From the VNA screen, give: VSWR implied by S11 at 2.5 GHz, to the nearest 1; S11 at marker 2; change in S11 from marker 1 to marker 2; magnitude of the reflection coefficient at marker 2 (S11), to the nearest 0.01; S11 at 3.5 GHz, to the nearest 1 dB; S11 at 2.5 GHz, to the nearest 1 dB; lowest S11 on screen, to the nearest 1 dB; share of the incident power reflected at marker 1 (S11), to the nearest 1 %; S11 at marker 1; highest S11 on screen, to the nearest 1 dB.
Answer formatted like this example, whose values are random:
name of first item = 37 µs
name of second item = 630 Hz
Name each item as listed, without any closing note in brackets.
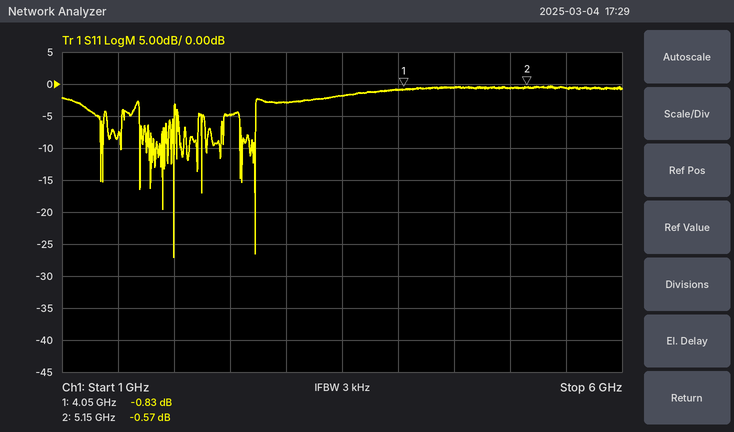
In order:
VSWR implied by S11 at 2.5 GHz, to the nearest 1 = 4
S11 at marker 2 = -0.57 dB
change in S11 from marker 1 to marker 2 = 0.26 dB
magnitude of the reflection coefficient at marker 2 (S11), to the nearest 0.01 = 0.94
S11 at 3.5 GHz, to the nearest 1 dB = -2 dB
S11 at 2.5 GHz, to the nearest 1 dB = -5 dB
lowest S11 on screen, to the nearest 1 dB = -27 dB
share of the incident power reflected at marker 1 (S11), to the nearest 1 % = 83 %
S11 at marker 1 = -0.83 dB
highest S11 on screen, to the nearest 1 dB = 0 dB
